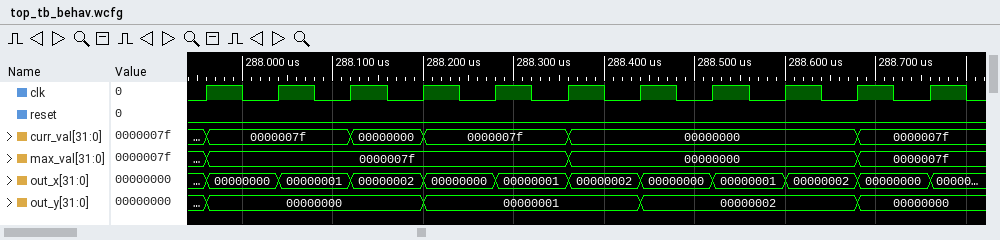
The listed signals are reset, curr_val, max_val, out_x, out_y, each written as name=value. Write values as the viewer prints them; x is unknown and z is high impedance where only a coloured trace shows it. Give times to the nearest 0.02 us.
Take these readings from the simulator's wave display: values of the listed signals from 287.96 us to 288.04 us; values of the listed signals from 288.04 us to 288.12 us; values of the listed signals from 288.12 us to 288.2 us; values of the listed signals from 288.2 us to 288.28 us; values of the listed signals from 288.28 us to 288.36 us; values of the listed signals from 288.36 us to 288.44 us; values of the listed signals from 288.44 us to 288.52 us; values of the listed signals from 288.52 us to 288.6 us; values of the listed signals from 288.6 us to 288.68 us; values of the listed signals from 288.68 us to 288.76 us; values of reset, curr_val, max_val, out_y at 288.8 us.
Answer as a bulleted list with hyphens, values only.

- reset=0, curr_val=0000007f, max_val=0000007f, out_x=00000000, out_y=00000000
- reset=0, curr_val=0000007f, max_val=0000007f, out_x=00000001, out_y=00000000
- reset=0, curr_val=00000000, max_val=0000007f, out_x=00000002, out_y=00000000
- reset=0, curr_val=0000007f, max_val=0000007f, out_x=00000000, out_y=00000001
- reset=0, curr_val=0000007f, max_val=0000007f, out_x=00000001, out_y=00000001
- reset=0, curr_val=00000000, max_val=00000000, out_x=00000002, out_y=00000001
- reset=0, curr_val=00000000, max_val=00000000, out_x=00000000, out_y=00000002
- reset=0, curr_val=00000000, max_val=00000000, out_x=00000001, out_y=00000002
- reset=0, curr_val=00000000, max_val=00000000, out_x=00000002, out_y=00000002
- reset=0, curr_val=0000007f, max_val=0000007f, out_x=00000000, out_y=00000000
- reset=0, curr_val=0000007f, max_val=0000007f, out_y=00000000
